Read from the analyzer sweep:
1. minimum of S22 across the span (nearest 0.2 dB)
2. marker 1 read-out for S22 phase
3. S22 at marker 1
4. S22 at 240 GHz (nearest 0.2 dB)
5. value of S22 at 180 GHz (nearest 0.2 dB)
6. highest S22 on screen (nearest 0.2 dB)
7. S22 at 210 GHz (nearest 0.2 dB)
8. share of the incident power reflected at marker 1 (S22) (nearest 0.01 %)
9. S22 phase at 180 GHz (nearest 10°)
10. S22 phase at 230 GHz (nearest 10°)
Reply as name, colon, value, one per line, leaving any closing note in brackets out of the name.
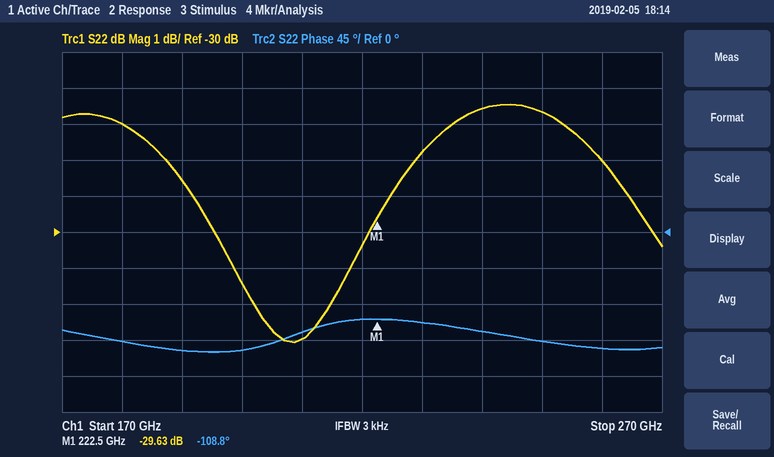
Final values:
minimum of S22 across the span: -33.0 dB
marker 1 read-out for S22 phase: -108.8°
S22 at marker 1: -29.63 dB
S22 at 240 GHz: -26.6 dB
value of S22 at 180 GHz: -27.0 dB
highest S22 on screen: -26.4 dB
S22 at 210 GHz: -33.0 dB
share of the incident power reflected at marker 1 (S22): 0.11 %
S22 phase at 180 GHz: -140°
S22 phase at 230 GHz: -110°
